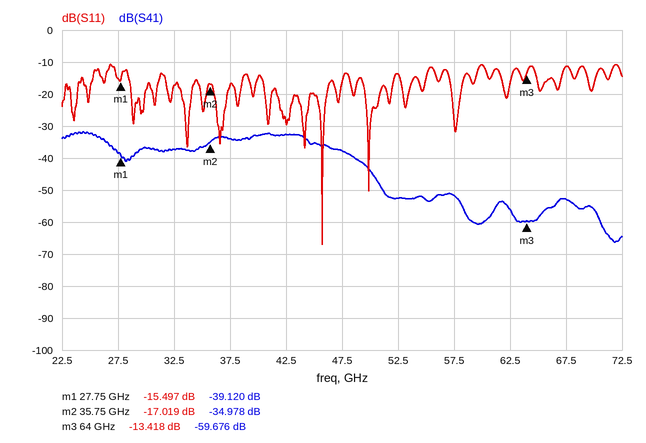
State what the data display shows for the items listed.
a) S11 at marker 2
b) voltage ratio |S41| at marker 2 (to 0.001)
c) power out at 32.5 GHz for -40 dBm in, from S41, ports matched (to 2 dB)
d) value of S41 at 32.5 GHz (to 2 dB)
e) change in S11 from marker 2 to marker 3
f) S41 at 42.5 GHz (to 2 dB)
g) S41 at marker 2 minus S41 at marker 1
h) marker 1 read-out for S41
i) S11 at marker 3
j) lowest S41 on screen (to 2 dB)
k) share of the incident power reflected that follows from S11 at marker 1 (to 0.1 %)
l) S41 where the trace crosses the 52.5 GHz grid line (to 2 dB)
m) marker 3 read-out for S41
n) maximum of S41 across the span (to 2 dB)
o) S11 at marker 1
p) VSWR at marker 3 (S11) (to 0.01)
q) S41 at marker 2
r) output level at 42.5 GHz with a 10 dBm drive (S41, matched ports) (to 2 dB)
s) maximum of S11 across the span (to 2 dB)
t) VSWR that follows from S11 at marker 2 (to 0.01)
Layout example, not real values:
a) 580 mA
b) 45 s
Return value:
a) -17.019 dB
b) 0.018
c) -78 dBm
d) -38 dB
e) 3.601 dB
f) -32 dB
g) 4.142 dB
h) -39.120 dB
i) -13.418 dB
j) -66 dB
k) 2.8 %
l) -52 dB
m) -59.676 dB
n) -32 dB
o) -15.497 dB
p) 1.54
q) -34.978 dB
r) -22 dBm
s) -10 dB
t) 1.33
